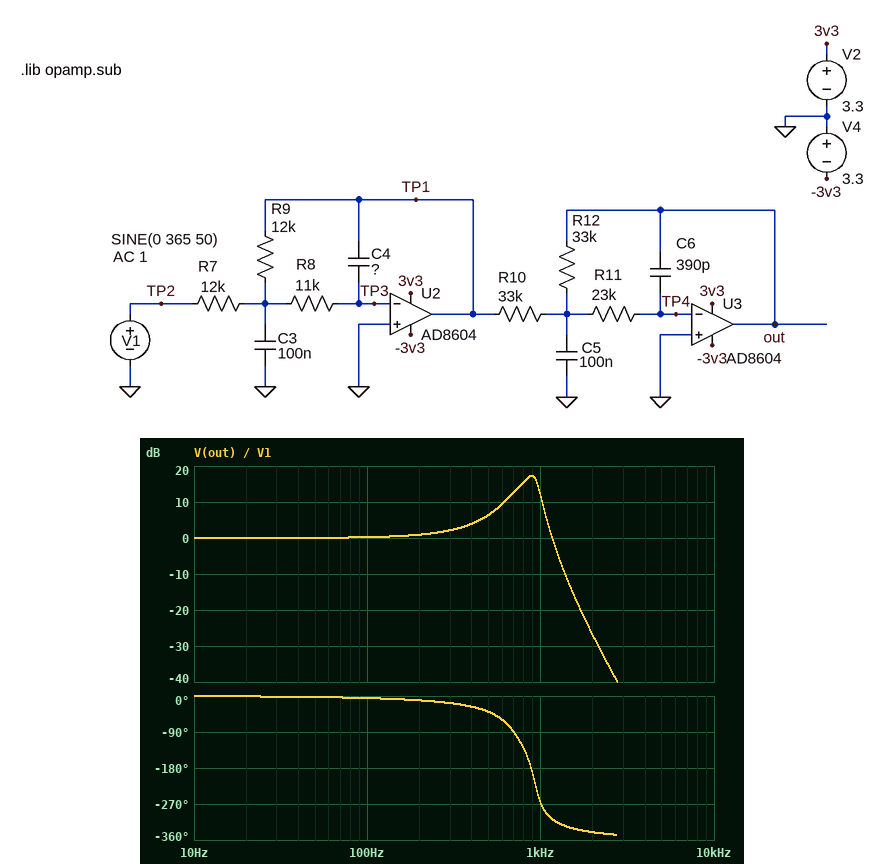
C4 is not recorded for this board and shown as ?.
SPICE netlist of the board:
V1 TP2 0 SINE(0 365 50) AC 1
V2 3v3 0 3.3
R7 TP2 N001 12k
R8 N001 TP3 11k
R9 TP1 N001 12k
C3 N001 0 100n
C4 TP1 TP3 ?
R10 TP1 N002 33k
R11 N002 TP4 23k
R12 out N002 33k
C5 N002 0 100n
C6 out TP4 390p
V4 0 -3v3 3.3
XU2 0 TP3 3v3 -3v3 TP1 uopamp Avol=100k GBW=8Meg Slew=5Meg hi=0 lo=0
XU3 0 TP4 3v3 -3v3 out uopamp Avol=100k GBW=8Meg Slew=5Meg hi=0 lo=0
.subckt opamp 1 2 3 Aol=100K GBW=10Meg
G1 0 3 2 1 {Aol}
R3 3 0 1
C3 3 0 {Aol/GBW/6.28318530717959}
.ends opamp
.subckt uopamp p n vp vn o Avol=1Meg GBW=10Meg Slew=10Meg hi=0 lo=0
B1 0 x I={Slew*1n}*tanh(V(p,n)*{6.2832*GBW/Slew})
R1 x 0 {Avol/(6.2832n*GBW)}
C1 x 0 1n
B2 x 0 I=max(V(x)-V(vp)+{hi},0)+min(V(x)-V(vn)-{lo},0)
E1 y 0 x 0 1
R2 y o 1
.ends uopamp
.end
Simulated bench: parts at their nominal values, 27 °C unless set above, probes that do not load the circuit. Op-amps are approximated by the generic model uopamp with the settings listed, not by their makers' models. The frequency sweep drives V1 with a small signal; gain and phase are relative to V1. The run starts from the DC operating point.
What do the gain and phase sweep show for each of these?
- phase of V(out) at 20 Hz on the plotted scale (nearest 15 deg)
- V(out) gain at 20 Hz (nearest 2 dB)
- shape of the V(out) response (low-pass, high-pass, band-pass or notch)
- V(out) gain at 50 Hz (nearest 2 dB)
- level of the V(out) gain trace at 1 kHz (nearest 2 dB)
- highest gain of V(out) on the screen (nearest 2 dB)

0 deg
0 dB
band-pass
0 dB
12 dB
18 dB
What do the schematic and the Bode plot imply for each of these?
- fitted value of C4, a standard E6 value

3.3 nF
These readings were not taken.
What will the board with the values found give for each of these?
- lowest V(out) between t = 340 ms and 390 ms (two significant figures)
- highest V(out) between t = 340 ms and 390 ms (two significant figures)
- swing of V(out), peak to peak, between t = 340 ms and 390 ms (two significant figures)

-3.3 V
3.3 V
6.6 V
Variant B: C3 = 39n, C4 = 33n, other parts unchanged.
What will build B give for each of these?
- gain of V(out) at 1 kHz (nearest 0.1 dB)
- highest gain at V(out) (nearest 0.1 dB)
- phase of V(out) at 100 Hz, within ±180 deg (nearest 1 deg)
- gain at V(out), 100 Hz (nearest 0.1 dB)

-7.4 dB
0 dB
-38 deg
-1.3 dB
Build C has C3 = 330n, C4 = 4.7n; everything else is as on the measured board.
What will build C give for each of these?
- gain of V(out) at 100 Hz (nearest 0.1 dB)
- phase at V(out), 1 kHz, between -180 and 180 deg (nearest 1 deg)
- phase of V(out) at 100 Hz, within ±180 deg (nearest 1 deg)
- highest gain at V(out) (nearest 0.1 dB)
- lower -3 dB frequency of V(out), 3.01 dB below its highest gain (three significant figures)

0.8 dB
57 deg
-7 deg
10.4 dB
278 Hz
